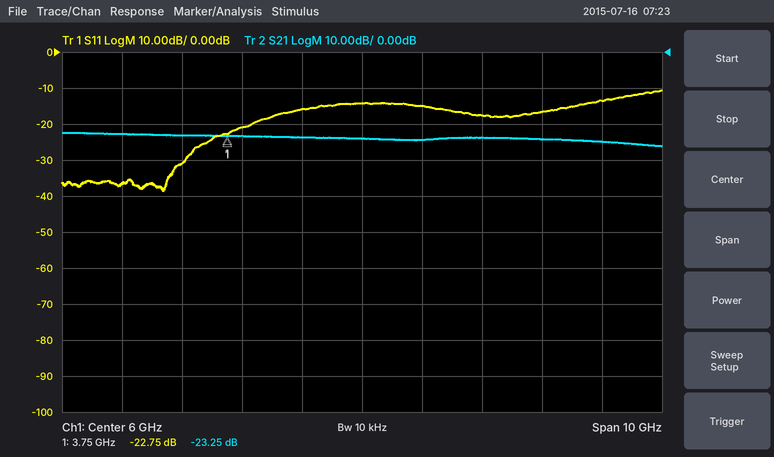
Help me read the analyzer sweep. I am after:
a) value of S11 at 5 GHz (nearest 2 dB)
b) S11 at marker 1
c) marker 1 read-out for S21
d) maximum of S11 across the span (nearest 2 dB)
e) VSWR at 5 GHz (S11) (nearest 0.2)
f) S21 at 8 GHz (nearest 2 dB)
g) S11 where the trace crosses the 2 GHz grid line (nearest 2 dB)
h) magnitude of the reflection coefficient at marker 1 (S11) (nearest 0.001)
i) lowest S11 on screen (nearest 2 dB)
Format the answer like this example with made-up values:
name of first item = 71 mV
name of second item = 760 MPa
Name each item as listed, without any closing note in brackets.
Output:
value of S11 at 5 GHz = -16 dB
S11 at marker 1 = -22.75 dB
marker 1 read-out for S21 = -23.25 dB
maximum of S11 across the span = -10 dB
VSWR at 5 GHz (S11) = 1.4
S21 at 8 GHz = -24 dB
S11 where the trace crosses the 2 GHz grid line = -36 dB
magnitude of the reflection coefficient at marker 1 (S11) = 0.073
lowest S11 on screen = -38 dB
